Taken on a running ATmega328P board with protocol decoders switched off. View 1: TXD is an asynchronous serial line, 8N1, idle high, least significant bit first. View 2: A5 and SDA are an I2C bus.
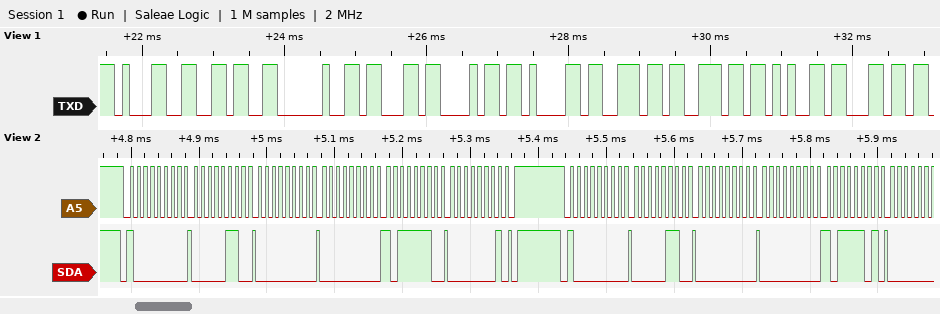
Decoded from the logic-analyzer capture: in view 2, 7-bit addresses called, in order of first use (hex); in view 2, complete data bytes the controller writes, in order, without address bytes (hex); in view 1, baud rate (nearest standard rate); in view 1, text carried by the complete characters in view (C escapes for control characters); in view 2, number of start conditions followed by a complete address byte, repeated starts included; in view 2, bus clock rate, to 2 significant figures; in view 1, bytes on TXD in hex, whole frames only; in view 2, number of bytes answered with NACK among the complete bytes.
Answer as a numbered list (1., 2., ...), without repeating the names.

1. 0x40
2. 06 00 00 BE 01 06 00 00 BD
3. 9600 baud
4. "16 channel"
5. 2
6. 100 kHz
7. 31 36 20 63 68 61 6E 6E 65 6C
8. 0
